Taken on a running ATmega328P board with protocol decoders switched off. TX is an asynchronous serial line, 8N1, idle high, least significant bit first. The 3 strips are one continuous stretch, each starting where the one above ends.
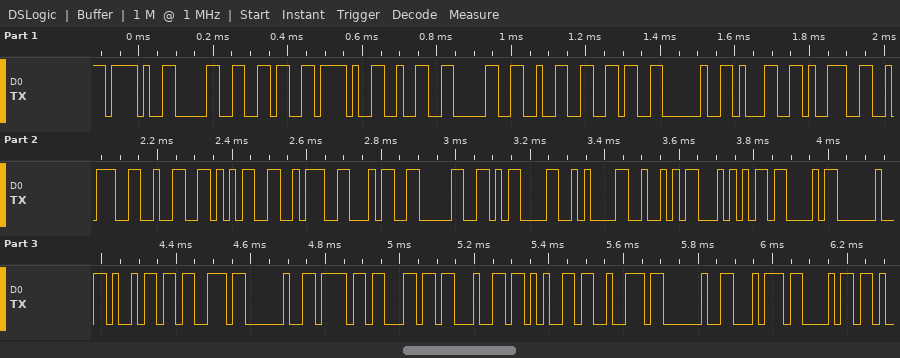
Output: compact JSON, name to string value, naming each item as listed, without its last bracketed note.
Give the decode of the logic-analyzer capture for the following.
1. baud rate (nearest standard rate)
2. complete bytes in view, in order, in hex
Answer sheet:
{"baud rate": "57600 baud", "complete bytes in view, in order, in hex": "2F 30 36 2F 32 30 32 36 20 31 39 3A 32 35 3A 34 30 0D 0A 52 54 43 20 69 73 20 6F 6C 64 65 72 20 74 68"}
